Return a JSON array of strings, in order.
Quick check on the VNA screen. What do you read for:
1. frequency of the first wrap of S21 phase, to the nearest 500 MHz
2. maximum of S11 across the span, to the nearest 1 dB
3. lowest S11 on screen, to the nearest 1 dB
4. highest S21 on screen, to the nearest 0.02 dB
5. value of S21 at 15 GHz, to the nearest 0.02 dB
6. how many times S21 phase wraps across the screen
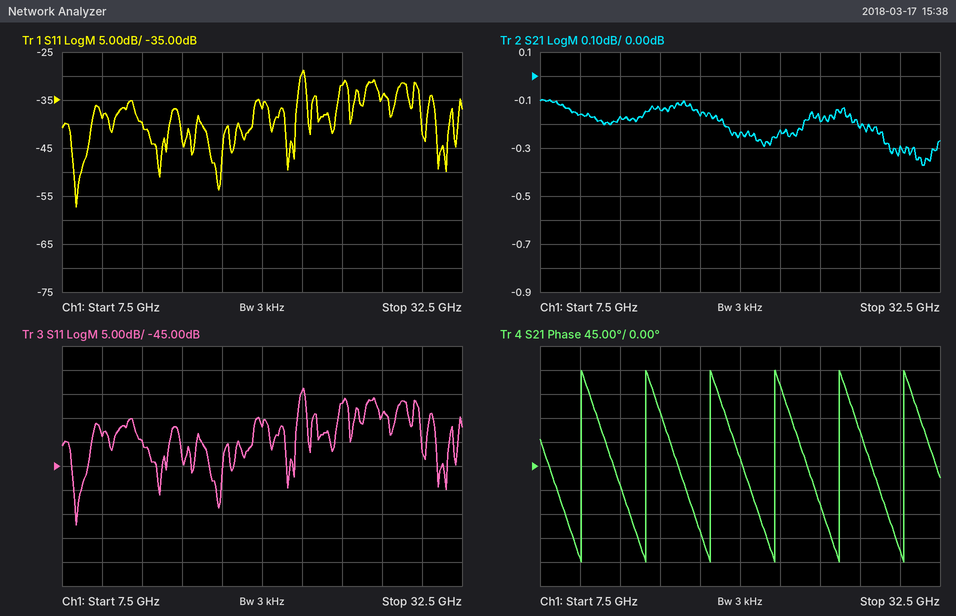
["10.0 GHz", "-29 dB", "-57 dB", "-0.10 dB", "-0.14 dB", "6"]
